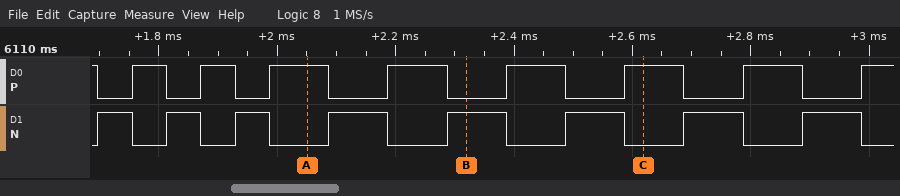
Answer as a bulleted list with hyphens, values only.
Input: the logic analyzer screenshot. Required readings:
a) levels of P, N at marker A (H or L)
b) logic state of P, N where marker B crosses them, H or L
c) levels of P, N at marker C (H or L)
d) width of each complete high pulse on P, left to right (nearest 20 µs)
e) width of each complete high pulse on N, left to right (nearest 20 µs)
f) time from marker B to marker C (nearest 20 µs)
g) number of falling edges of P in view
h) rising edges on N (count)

- P=H, N=L
- P=L, N=H
- P=H, N=L
- 60 µs, 60 µs, 100 µs, 100 µs, 100 µs, 100 µs, 100 µs
- 60 µs, 60 µs, 60 µs, 100 µs, 100 µs, 100 µs, 100 µs, 100 µs
- 300 µs
- 8
- 8
